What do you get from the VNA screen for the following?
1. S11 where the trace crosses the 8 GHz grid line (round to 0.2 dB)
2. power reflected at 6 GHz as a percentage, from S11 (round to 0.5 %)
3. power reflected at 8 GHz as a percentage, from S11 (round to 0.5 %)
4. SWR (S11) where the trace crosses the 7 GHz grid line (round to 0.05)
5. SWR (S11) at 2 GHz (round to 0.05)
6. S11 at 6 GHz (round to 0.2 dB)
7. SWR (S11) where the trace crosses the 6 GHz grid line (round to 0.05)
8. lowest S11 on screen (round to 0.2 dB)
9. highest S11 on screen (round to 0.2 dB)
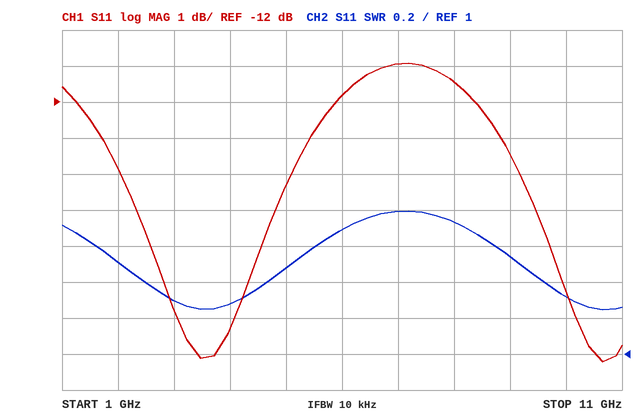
-11.4 dB
6.5 %
7.0 %
1.80
1.50
-11.8 dB
1.70
-19.2 dB
-11.0 dB
